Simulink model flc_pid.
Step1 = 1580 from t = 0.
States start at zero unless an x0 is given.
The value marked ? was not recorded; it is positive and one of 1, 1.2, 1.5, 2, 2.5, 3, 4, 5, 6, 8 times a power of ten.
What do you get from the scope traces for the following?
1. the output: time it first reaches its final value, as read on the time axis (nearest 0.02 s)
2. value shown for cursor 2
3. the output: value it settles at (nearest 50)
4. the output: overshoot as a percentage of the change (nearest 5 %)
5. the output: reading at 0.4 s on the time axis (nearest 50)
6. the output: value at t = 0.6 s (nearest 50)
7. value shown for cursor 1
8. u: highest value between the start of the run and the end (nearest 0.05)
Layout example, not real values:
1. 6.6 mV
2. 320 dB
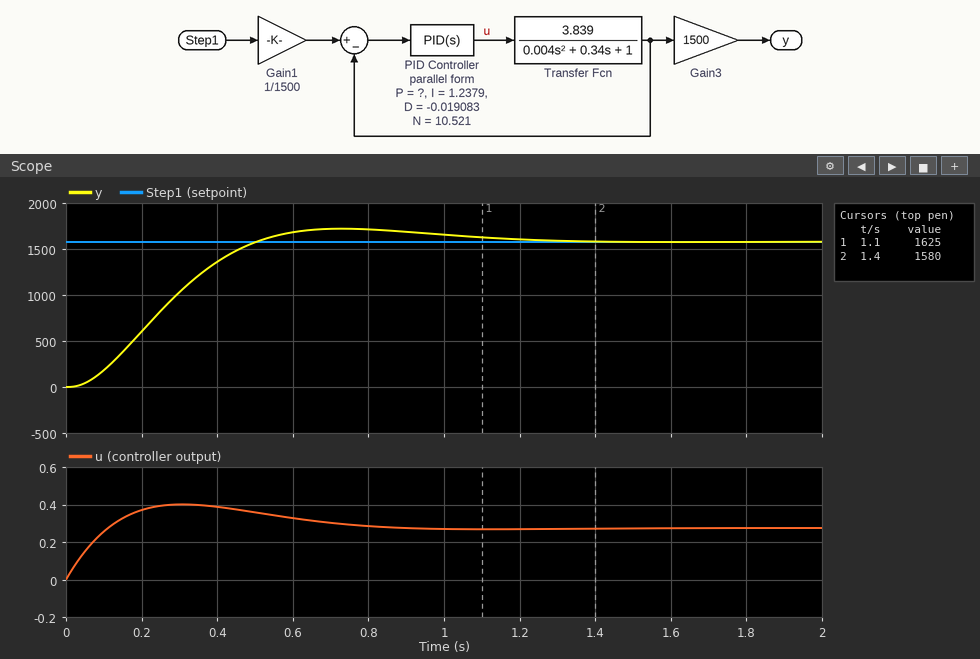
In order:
1. 0.50 s
2. 1580
3. 1600
4. 10 %
5. 1350
6. 1700
7. 1625
8. 0.40
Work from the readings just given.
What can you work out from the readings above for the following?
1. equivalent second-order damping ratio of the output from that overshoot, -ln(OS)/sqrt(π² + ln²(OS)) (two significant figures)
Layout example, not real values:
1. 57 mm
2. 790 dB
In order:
1. 0.59
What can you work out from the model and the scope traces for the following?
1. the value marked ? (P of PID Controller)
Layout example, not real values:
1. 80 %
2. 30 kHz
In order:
1. 0.2
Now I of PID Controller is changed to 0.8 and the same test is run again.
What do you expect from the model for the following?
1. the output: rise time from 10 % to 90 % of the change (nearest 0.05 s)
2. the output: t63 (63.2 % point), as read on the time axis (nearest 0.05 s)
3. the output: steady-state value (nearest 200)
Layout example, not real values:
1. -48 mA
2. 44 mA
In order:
1. 0.50 s
2. 0.35 s
3. 1600
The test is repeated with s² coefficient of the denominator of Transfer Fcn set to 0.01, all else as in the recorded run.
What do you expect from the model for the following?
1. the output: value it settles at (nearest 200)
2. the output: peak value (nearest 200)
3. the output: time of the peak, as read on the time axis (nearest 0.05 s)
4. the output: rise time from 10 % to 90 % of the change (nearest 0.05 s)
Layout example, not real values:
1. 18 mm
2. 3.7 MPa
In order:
1. 1600
2. 1800
3. 0.70 s
4. 0.30 s
